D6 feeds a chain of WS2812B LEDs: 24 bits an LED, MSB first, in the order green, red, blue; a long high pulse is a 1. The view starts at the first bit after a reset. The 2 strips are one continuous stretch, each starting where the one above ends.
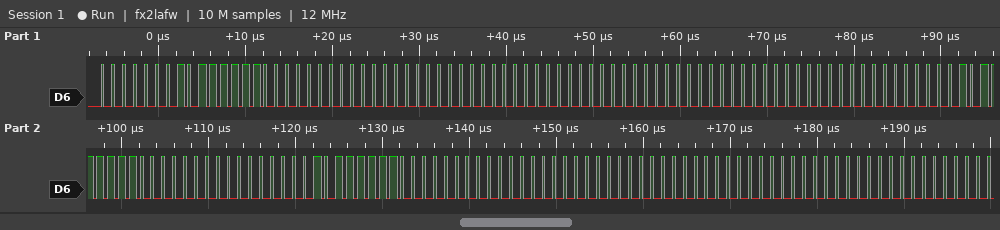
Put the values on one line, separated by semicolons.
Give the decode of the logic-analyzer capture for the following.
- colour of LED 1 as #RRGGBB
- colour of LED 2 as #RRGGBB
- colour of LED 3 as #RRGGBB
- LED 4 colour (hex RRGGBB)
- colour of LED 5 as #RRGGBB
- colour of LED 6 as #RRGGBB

#7E0100; #000000; #000000; #7E0100; #7E0100; #000000
